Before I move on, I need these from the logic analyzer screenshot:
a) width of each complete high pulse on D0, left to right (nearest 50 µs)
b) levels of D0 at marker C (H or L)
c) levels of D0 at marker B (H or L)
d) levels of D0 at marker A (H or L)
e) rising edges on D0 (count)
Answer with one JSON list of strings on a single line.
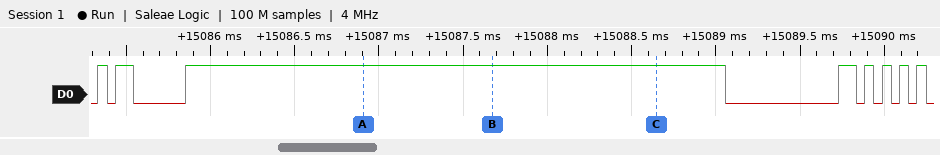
["50 µs, 100 µs, 3200 µs, 100 µs, 50 µs, 50 µs, 50 µs, 50 µs", "D0=H", "D0=H", "D0=H", "8"]
